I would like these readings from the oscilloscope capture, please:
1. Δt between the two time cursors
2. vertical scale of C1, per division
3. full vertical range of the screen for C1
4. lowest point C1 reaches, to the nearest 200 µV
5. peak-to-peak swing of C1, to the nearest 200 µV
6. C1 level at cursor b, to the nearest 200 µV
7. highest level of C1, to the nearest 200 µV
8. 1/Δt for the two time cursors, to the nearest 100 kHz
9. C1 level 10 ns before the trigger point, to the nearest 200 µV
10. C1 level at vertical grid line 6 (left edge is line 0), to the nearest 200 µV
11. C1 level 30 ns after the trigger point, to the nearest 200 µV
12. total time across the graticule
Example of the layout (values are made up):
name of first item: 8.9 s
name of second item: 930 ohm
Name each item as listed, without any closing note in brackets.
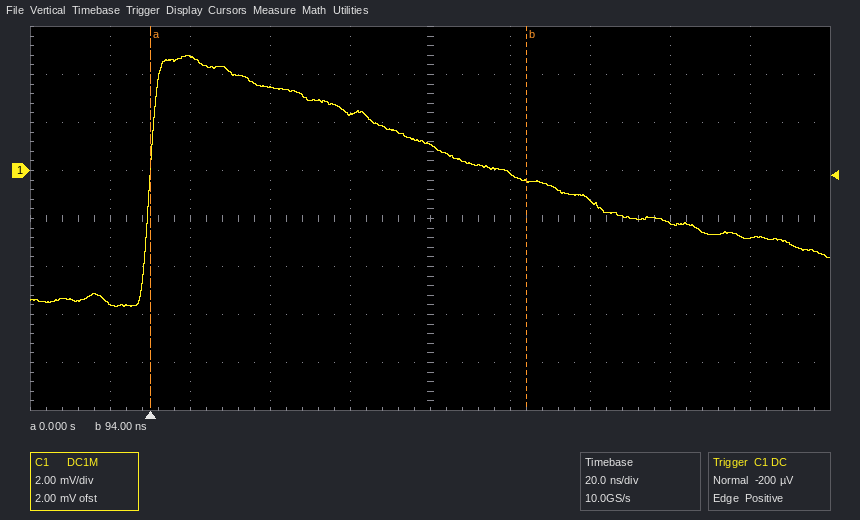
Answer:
Δt between the two time cursors: 94 ns
vertical scale of C1, per division: 2 mV
full vertical range of the screen for C1: 16 mV
lowest point C1 reaches, to the nearest 200 µV: -5.6 mV
peak-to-peak swing of C1, to the nearest 200 µV: 10.4 mV
C1 level at cursor b, to the nearest 200 µV: -400 µV
highest level of C1, to the nearest 200 µV: 4.8 mV
1/Δt for the two time cursors, to the nearest 100 kHz: 10.6 MHz
C1 level 10 ns before the trigger point, to the nearest 200 µV: -5.6 mV
C1 level at vertical grid line 6 (left edge is line 0), to the nearest 200 µV: -200 µV
C1 level 30 ns after the trigger point, to the nearest 200 µV: 3.4 mV
total time across the graticule: 200 ns
